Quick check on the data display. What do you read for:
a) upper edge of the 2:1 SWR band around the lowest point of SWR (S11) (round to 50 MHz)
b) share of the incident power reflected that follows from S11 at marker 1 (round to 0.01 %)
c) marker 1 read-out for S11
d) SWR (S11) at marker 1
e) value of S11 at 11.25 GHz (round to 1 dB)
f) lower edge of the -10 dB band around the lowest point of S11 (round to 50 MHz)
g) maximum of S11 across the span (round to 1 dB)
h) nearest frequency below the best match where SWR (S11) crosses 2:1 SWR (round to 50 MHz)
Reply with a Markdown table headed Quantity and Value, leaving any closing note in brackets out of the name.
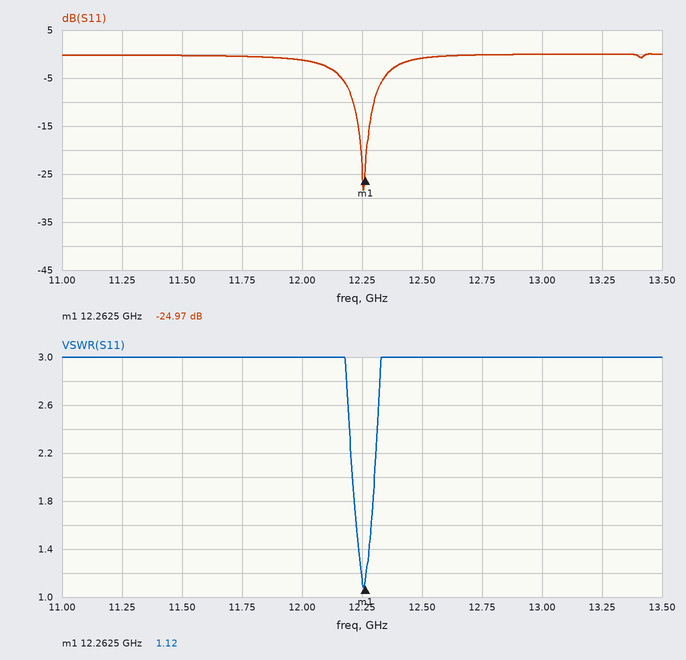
| Quantity | Value |
|---|---|
| upper edge of the 2:1 SWR band around the lowest point of SWR (S11) | 12.30 GHz |
| share of the incident power reflected that follows from S11 at marker 1 | 0.32 % |
| marker 1 read-out for S11 | -24.97 dB |
| SWR (S11) at marker 1 | 1.12 |
| value of S11 at 11.25 GHz | 0 dB |
| lower edge of the -10 dB band around the lowest point of S11 | 12.20 GHz |
| maximum of S11 across the span | 0 dB |
| nearest frequency below the best match where SWR (S11) crosses 2:1 SWR | 12.20 GHz |
